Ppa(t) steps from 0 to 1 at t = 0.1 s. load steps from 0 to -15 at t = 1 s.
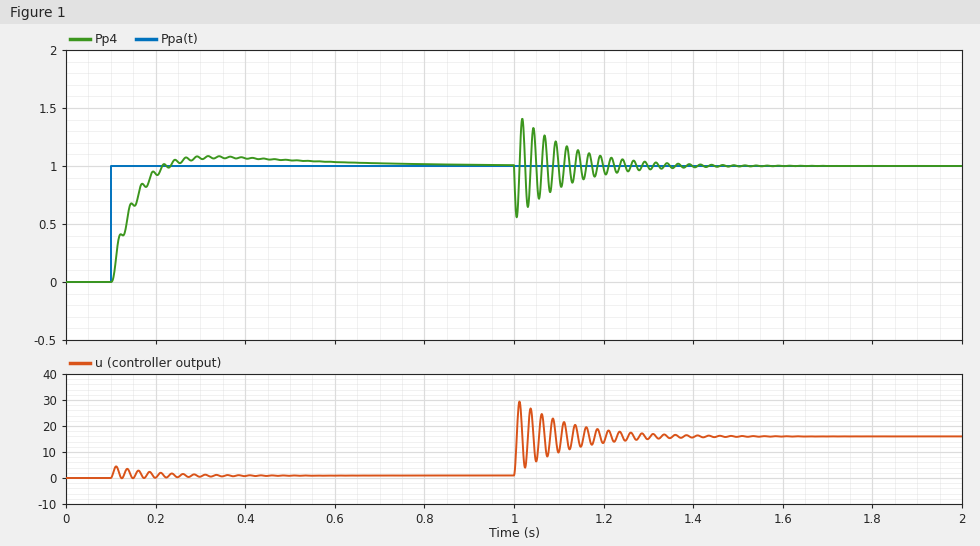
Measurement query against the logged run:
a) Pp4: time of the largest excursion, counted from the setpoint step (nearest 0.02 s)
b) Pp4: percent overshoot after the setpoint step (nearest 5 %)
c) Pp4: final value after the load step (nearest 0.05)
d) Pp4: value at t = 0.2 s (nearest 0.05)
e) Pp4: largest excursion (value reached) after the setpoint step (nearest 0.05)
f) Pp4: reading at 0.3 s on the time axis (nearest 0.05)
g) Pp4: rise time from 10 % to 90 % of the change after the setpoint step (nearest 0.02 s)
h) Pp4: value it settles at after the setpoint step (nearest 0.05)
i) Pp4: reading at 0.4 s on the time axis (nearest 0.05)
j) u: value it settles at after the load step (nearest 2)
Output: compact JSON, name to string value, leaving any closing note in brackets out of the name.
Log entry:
{"Pp4: time of the largest excursion, counted from the setpoint step": "0.22 s", "Pp4: percent overshoot after the setpoint step": "10 %", "Pp4: final value after the load step": "1.00", "Pp4: value at t = 0.2 s": "0.95", "Pp4: largest excursion (value reached) after the setpoint step": "1.10", "Pp4: reading at 0.3 s on the time axis": "1.05", "Pp4: rise time from 10 % to 90 % of the change after the setpoint step": "0.08 s", "Pp4: value it settles at after the setpoint step": "1.00", "Pp4: reading at 0.4 s on the time axis": "1.05", "u: value it settles at after the load step": "16"}
